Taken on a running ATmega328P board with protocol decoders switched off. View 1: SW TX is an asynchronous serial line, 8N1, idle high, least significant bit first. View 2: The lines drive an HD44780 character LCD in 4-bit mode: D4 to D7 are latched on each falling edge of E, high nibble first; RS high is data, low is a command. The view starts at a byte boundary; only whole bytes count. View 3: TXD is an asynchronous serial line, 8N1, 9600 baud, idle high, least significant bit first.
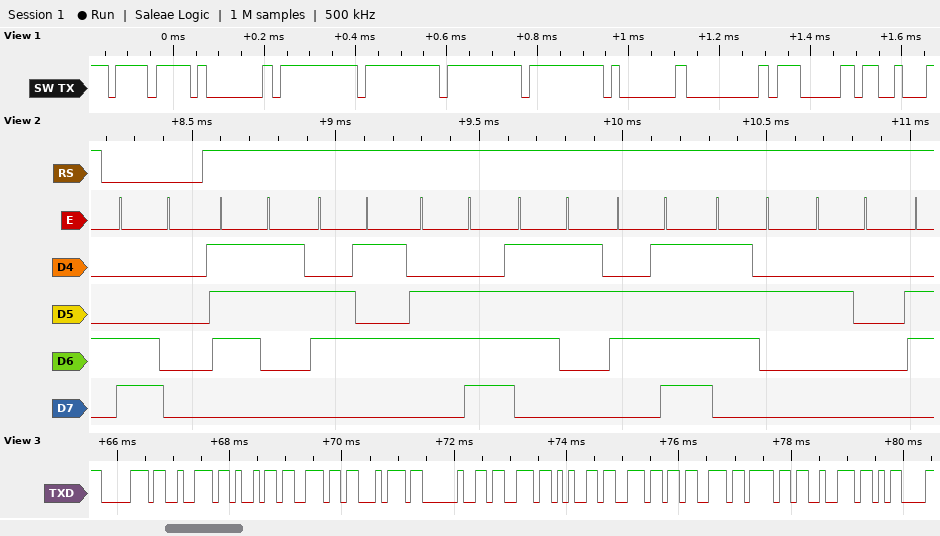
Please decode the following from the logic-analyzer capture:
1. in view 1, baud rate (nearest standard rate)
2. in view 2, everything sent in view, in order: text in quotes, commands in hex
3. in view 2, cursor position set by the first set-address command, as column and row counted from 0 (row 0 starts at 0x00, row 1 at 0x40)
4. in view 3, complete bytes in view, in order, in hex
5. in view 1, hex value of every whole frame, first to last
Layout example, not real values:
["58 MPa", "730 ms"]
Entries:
["57600 baud", "0xC0 \"sensor \"", "column 0, row 1", "70 72 69 6E 74 20 73 65 6E 73 6F 72 0D", "0xEF 0x01 0xFF 0xFF 0xFF 0xFF 0x01 0x00 0x07 0x13"]
